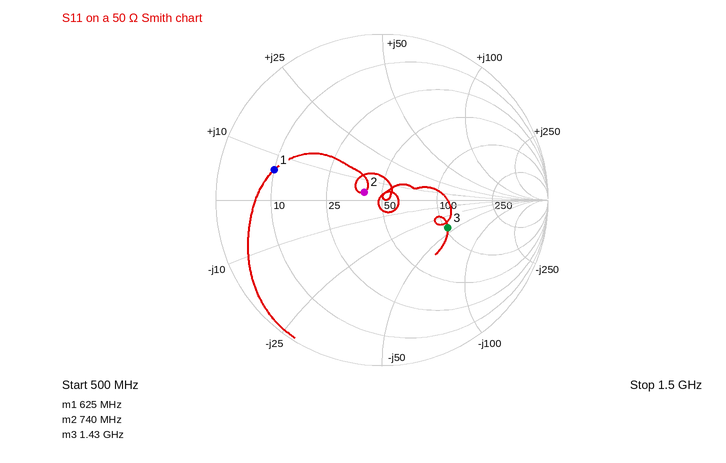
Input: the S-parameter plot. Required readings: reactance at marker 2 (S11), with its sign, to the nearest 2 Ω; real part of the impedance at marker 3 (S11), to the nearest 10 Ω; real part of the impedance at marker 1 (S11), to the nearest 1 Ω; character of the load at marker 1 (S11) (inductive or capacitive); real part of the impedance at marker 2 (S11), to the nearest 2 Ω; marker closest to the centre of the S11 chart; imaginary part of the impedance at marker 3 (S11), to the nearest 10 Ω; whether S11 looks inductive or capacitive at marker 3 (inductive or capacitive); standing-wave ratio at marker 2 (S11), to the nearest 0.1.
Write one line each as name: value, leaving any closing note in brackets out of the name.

reactance at marker 2 (S11), with its sign, to the nearest 2 Ω: +4 Ω
real part of the impedance at marker 3 (S11), to the nearest 10 Ω: 100 Ω
real part of the impedance at marker 1 (S11), to the nearest 1 Ω: 10 Ω
character of the load at marker 1 (S11): inductive
real part of the impedance at marker 2 (S11), to the nearest 2 Ω: 40 Ω
marker closest to the centre of the S11 chart: marker 2
imaginary part of the impedance at marker 3 (S11), to the nearest 10 Ω: -40 Ω
whether S11 looks inductive or capacitive at marker 3: capacitive
standing-wave ratio at marker 2 (S11), to the nearest 0.1: 1.3
